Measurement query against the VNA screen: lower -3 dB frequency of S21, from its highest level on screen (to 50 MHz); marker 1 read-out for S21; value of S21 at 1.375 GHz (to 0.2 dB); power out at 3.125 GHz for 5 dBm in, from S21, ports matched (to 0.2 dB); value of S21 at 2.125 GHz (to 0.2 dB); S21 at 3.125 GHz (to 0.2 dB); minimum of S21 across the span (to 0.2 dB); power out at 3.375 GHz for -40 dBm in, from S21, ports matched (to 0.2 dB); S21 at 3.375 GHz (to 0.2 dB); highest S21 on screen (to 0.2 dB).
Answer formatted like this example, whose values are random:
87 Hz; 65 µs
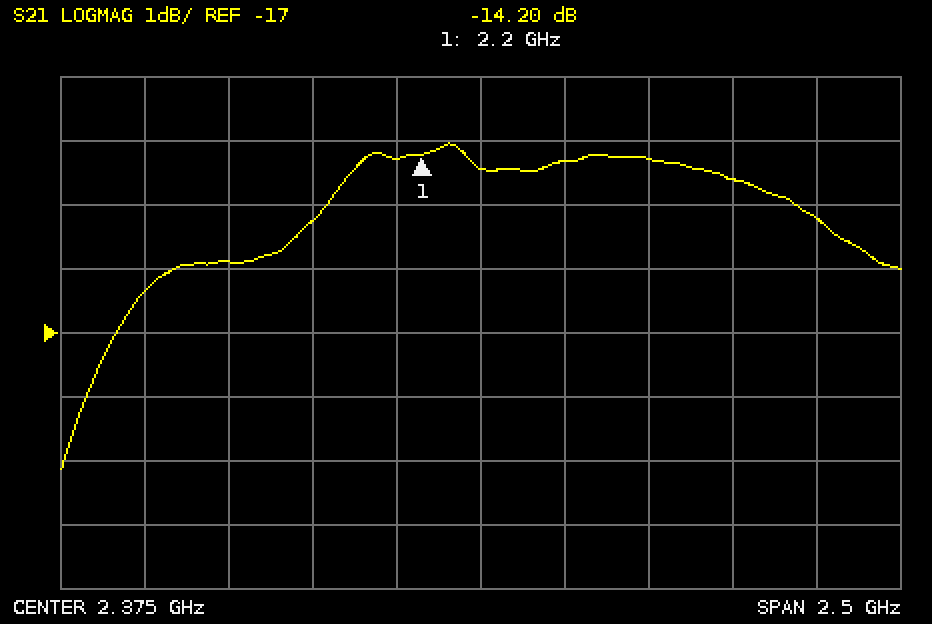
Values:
1.30 GHz; -14.20 dB; -16.4 dB; -9.6 dBm; -14.2 dB; -14.6 dB; -19.2 dB; -55.2 dBm; -15.2 dB; -14.0 dB
